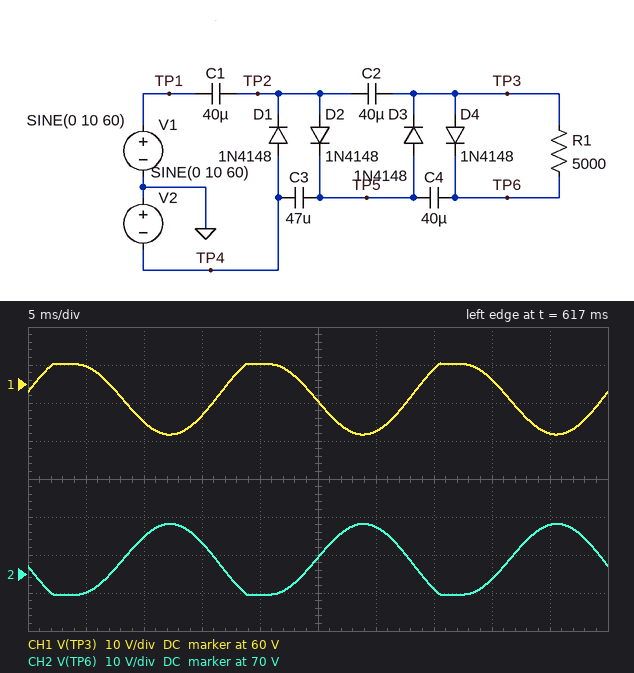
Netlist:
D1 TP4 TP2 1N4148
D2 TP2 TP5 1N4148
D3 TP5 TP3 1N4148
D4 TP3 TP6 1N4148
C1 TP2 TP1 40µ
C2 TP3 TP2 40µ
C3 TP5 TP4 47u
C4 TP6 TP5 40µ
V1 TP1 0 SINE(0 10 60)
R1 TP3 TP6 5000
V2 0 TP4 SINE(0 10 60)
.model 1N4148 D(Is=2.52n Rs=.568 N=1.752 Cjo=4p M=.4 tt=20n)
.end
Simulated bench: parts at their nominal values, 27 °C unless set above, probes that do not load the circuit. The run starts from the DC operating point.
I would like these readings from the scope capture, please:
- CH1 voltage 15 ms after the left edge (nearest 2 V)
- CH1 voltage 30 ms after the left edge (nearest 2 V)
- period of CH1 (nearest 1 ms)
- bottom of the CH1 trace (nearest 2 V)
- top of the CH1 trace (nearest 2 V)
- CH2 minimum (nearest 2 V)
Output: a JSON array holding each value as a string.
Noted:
["52 V", "48 V", "17 ms", "46 V", "66 V", "64 V"]
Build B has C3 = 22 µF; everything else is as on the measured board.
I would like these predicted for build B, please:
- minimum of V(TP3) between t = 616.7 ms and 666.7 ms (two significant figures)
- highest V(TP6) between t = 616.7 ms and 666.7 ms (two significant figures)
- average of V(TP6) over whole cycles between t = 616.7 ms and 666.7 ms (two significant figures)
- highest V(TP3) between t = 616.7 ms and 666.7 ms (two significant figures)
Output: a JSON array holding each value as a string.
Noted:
["46 V", "82 V", "72 V", "64 V"]
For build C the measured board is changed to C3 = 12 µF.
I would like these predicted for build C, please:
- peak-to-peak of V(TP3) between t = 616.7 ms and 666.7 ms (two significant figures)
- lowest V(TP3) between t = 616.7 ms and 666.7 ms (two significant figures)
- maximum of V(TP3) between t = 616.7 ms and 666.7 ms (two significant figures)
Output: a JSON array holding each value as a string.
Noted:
["18 V", "44 V", "63 V"]
